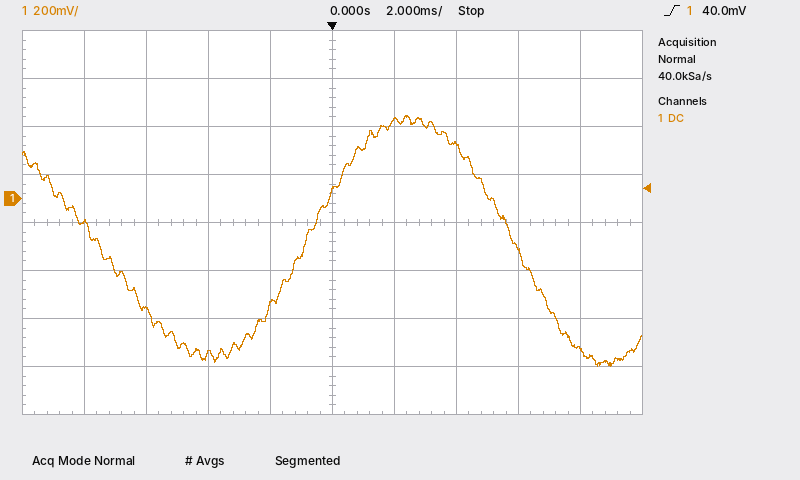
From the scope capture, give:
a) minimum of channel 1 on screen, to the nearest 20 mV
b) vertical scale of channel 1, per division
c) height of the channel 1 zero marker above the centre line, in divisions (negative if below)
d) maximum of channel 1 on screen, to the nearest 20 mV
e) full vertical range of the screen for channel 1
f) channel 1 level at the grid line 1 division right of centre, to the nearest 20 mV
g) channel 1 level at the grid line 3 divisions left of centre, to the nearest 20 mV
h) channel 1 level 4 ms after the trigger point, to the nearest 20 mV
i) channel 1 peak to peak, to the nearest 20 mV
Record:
-700 mV
200 mV
+0.5 div
340 mV
1.6 V
320 mV
-460 mV
220 mV
1.04 V
